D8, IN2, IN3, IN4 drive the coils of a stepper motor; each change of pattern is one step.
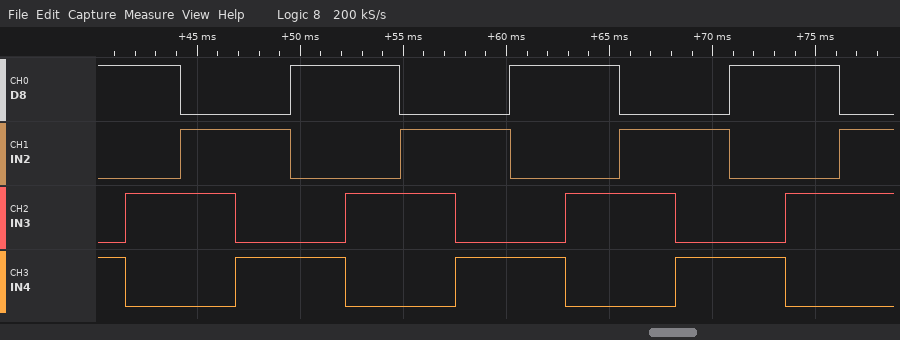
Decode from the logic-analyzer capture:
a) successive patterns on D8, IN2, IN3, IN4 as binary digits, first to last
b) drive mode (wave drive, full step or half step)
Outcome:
1001 1010 0110 0101 1001 1010 0110 0101 1001 1010 0110 0101 1001 1010 0110
full step
